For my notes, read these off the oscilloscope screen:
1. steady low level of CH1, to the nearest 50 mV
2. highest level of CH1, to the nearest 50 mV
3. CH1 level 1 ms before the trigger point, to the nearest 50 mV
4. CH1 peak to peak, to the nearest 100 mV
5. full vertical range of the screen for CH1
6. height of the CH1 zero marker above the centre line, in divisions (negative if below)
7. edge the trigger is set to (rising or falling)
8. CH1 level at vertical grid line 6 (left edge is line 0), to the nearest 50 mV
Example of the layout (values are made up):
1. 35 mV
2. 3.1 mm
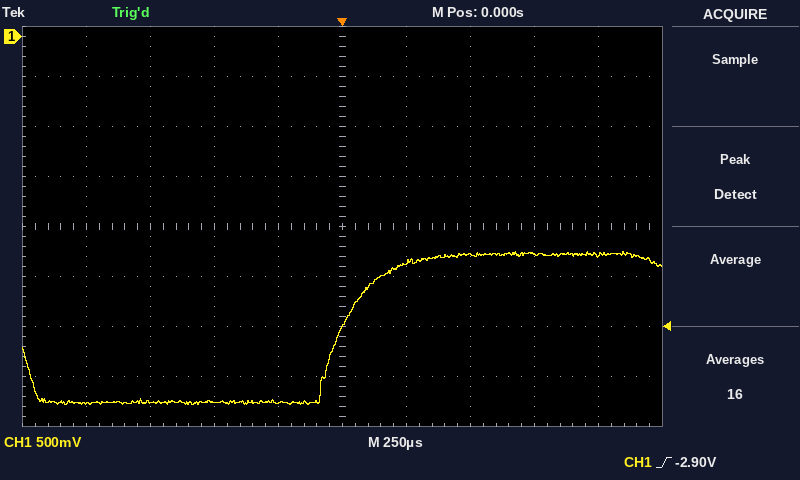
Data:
1. -3.65 V
2. -2.15 V
3. -3.65 V
4. 1.50 V
5. 4 V
6. +3.8 div
7. rising
8. -2.25 V
